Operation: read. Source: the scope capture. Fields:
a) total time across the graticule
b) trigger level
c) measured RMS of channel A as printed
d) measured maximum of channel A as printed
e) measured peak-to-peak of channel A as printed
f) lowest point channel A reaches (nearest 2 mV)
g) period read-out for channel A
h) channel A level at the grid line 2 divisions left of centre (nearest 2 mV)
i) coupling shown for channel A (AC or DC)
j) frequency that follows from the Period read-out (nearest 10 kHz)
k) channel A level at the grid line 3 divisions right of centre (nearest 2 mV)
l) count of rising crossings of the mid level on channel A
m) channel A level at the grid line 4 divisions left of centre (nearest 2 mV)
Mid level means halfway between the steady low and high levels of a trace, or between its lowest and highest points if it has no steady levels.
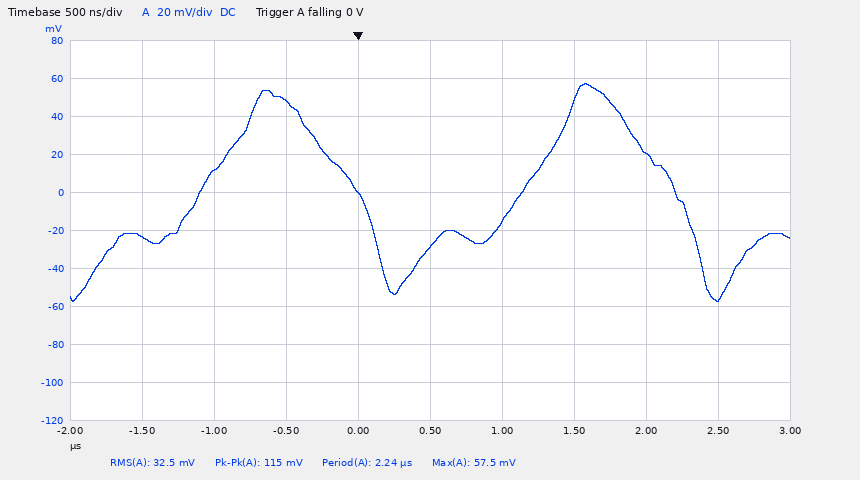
5 µs
0 V
32.5 mV
57.5 mV
115 mV
-58 mV
2.24 µs
48 mV
DC
450 kHz
20 mV
2
-24 mV
